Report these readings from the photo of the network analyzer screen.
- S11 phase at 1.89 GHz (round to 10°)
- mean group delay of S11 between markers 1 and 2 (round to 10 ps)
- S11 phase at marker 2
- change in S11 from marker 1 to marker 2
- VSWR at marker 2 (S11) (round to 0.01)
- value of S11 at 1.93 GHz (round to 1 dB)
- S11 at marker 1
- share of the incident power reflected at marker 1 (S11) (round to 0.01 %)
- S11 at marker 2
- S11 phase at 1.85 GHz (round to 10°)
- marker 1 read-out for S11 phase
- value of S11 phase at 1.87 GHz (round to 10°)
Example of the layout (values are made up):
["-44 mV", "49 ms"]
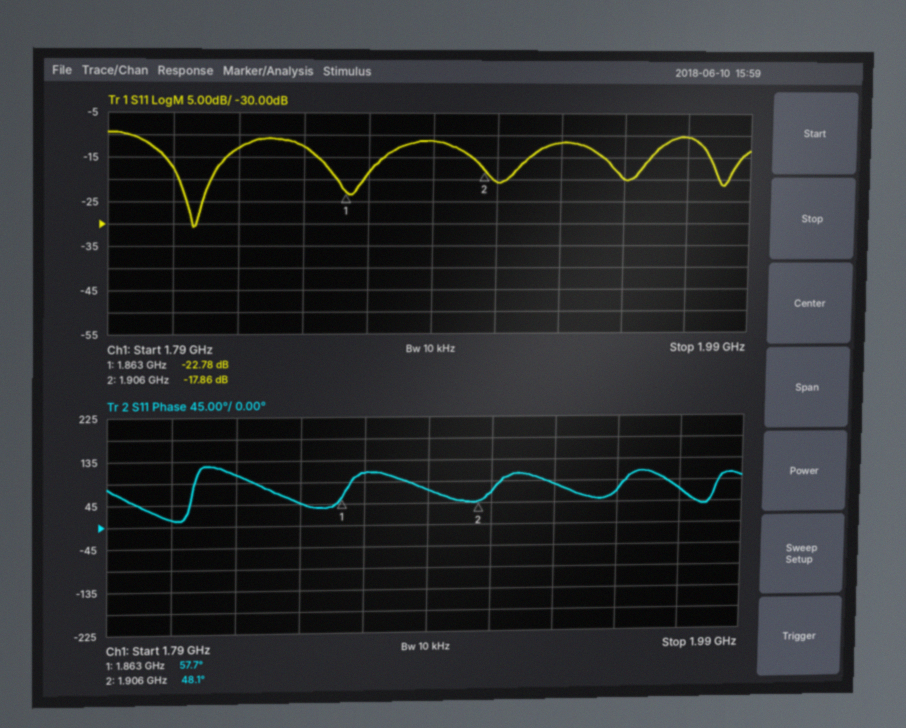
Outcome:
["70°", "620 ps", "48.1°", "4.92 dB", "1.29", "-12 dB", "-22.78 dB", "0.53 %", "-17.86 dB", "50°", "57.7°", "110°"]
